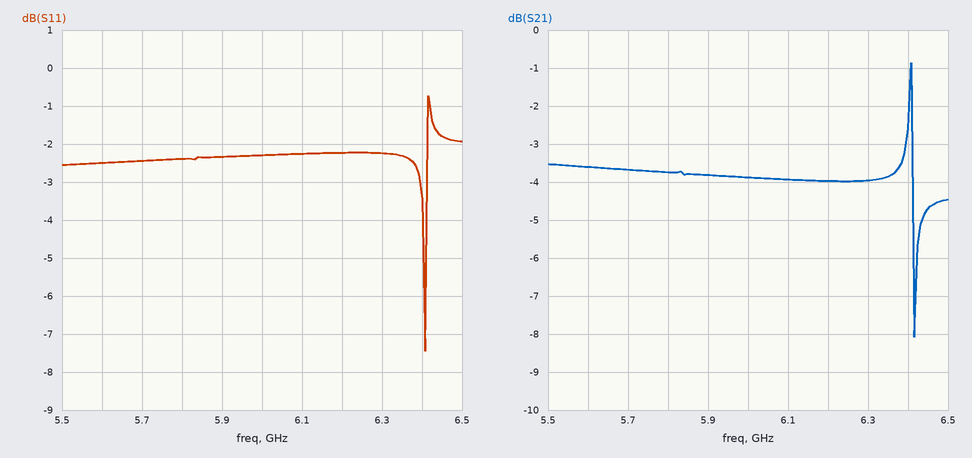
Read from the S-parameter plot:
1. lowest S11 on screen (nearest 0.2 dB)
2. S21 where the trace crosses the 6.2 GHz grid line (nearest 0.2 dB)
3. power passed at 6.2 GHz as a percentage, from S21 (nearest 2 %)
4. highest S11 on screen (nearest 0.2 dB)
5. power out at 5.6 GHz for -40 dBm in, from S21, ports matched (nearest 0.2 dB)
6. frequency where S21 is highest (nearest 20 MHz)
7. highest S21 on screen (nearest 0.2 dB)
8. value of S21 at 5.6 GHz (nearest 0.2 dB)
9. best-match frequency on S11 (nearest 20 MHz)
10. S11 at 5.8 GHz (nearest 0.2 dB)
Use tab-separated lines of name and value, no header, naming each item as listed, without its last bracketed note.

lowest S11 on screen	-7.4 dB
S21 where the trace crosses the 6.2 GHz grid line	-4.0 dB
power passed at 6.2 GHz as a percentage, from S21	40 %
highest S11 on screen	-0.8 dB
power out at 5.6 GHz for -40 dBm in, from S21, ports matched	-43.6 dBm
frequency where S21 is highest	6.40 GHz
highest S21 on screen	-0.8 dB
value of S21 at 5.6 GHz	-3.6 dB
best-match frequency on S11	6.40 GHz
S11 at 5.8 GHz	-2.4 dB
